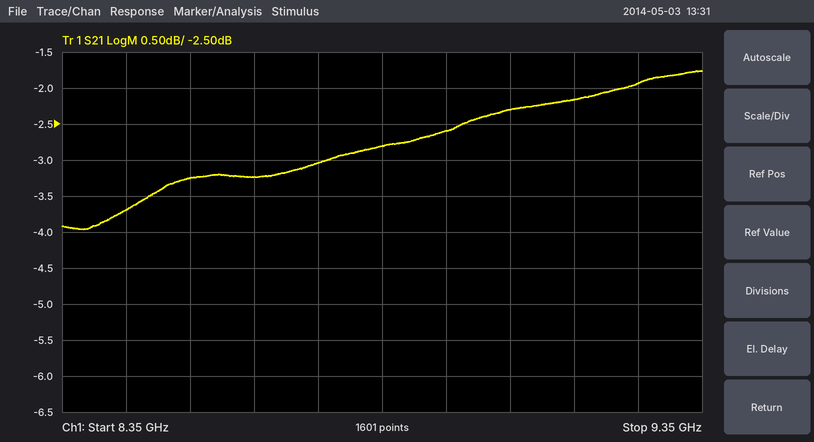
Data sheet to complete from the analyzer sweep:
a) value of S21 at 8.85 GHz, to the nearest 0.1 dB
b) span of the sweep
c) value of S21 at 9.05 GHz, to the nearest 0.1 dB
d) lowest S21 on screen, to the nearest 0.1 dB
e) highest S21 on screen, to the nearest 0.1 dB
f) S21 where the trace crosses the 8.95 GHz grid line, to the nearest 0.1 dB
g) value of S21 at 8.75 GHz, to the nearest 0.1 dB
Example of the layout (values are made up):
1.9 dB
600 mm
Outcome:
-2.8 dB
1 GHz
-2.3 dB
-4.0 dB
-1.8 dB
-2.6 dB
-3.0 dB
